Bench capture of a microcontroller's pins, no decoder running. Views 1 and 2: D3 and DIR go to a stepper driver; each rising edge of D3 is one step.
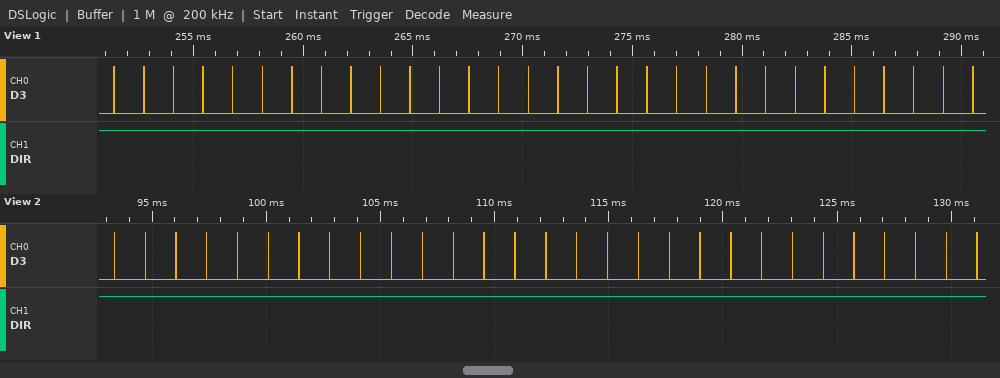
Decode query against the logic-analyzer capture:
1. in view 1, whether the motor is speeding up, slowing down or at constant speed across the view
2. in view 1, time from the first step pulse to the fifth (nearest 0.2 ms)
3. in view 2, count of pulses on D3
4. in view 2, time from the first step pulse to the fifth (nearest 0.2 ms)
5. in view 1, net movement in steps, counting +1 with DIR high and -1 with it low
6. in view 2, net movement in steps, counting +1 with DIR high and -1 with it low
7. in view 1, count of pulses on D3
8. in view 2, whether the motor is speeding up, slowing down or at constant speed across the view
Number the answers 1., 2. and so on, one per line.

1. constant speed
2. 5.4 ms
3. 29
4. 5.4 ms
5. +30
6. +29
7. 30
8. constant speed
